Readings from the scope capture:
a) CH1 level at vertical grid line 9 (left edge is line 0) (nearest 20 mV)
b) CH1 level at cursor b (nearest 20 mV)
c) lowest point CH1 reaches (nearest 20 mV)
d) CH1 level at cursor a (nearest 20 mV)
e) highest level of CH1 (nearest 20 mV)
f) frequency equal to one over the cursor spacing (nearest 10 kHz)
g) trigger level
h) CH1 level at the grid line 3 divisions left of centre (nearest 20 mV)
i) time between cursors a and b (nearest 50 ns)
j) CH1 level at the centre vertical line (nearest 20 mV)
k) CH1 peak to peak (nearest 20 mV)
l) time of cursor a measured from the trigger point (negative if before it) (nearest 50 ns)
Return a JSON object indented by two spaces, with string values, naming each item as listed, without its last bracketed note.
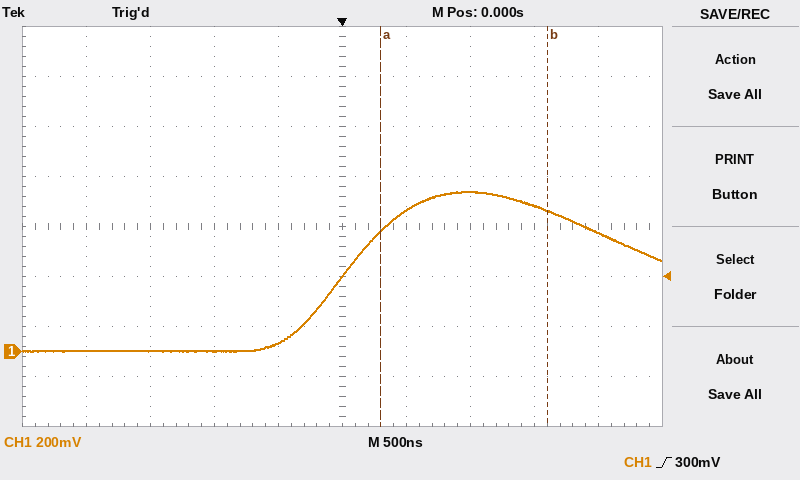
{
  "CH1 level at vertical grid line 9 (left edge is line 0)": "480 mV",
  "CH1 level at cursor b": "560 mV",
  "lowest point CH1 reaches": "0 mV",
  "CH1 level at cursor a": "480 mV",
  "highest level of CH1": "640 mV",
  "frequency equal to one over the cursor spacing": "770 kHz",
  "trigger level": "300 mV",
  "CH1 level at the grid line 3 divisions left of centre": "0 mV",
  "time between cursors a and b": "1.30 µs",
  "CH1 level at the centre vertical line": "300 mV",
  "CH1 peak to peak": "640 mV",
  "time of cursor a measured from the trigger point (negative if before it)": "+300 ns"
}
